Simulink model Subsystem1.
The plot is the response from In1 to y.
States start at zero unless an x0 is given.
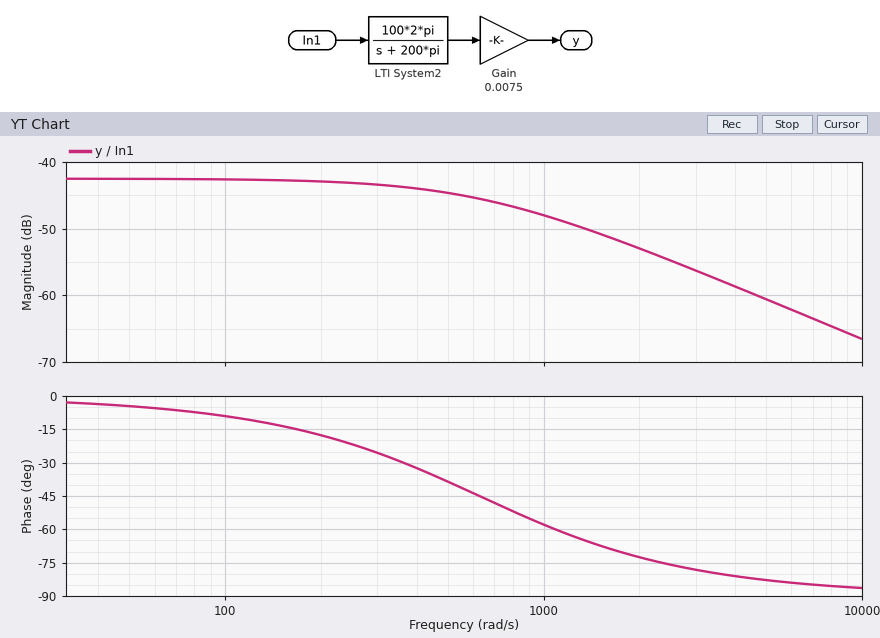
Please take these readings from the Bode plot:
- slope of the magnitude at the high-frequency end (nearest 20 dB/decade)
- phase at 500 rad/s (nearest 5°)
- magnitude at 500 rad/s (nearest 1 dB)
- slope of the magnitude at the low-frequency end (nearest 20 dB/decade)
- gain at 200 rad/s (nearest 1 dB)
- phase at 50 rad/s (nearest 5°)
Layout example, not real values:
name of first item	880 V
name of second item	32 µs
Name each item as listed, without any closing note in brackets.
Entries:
slope of the magnitude at the high-frequency end	-20 dB/decade
phase at 500 rad/s	-40°
magnitude at 500 rad/s	-45 dB
slope of the magnitude at the low-frequency end	0 dB/decade
gain at 200 rad/s	-43 dB
phase at 50 rad/s	-5°
